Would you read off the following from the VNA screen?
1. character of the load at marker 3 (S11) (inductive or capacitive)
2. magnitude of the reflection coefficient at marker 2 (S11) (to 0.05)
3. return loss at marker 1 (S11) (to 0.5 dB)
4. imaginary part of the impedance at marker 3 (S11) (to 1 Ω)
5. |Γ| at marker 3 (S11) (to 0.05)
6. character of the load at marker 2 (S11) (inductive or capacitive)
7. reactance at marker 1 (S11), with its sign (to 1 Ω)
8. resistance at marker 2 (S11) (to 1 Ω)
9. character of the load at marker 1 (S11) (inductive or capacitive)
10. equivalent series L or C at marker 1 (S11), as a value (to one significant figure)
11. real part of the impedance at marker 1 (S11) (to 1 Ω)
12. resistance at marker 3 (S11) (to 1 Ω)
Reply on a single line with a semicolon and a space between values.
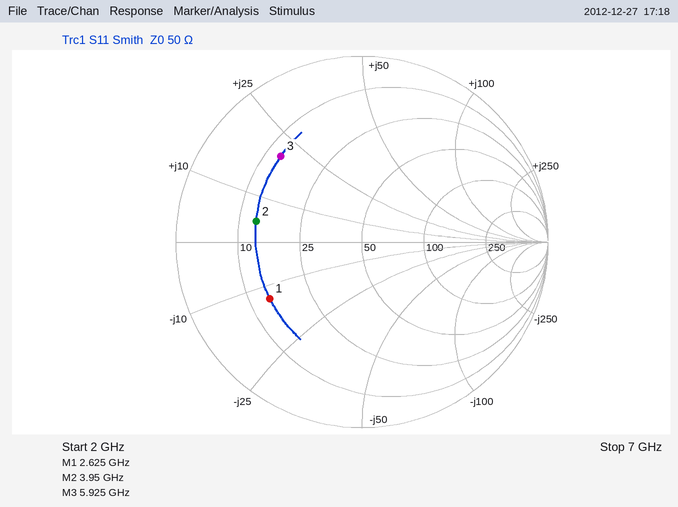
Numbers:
inductive; 0.60; 4.5 dB; +20 Ω; 0.65; inductive; -13 Ω; 13 Ω; capacitive; 5 pF; 14 Ω; 13 Ω
